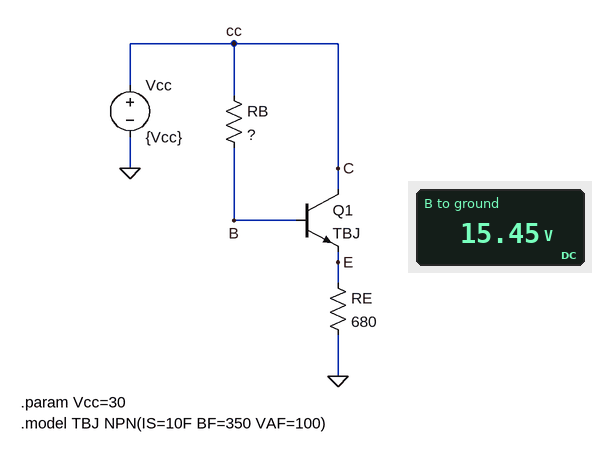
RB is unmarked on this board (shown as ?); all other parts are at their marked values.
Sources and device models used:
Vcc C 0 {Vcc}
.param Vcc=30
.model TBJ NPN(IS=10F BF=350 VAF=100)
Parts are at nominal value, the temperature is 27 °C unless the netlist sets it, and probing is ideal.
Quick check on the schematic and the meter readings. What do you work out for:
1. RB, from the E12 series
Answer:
270 kΩ
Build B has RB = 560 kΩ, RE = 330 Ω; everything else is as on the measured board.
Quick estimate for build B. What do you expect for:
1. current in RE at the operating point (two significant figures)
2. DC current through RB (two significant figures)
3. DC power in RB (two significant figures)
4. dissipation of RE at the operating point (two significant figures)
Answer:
18 mA
42 µA
970 µW
110 mW
